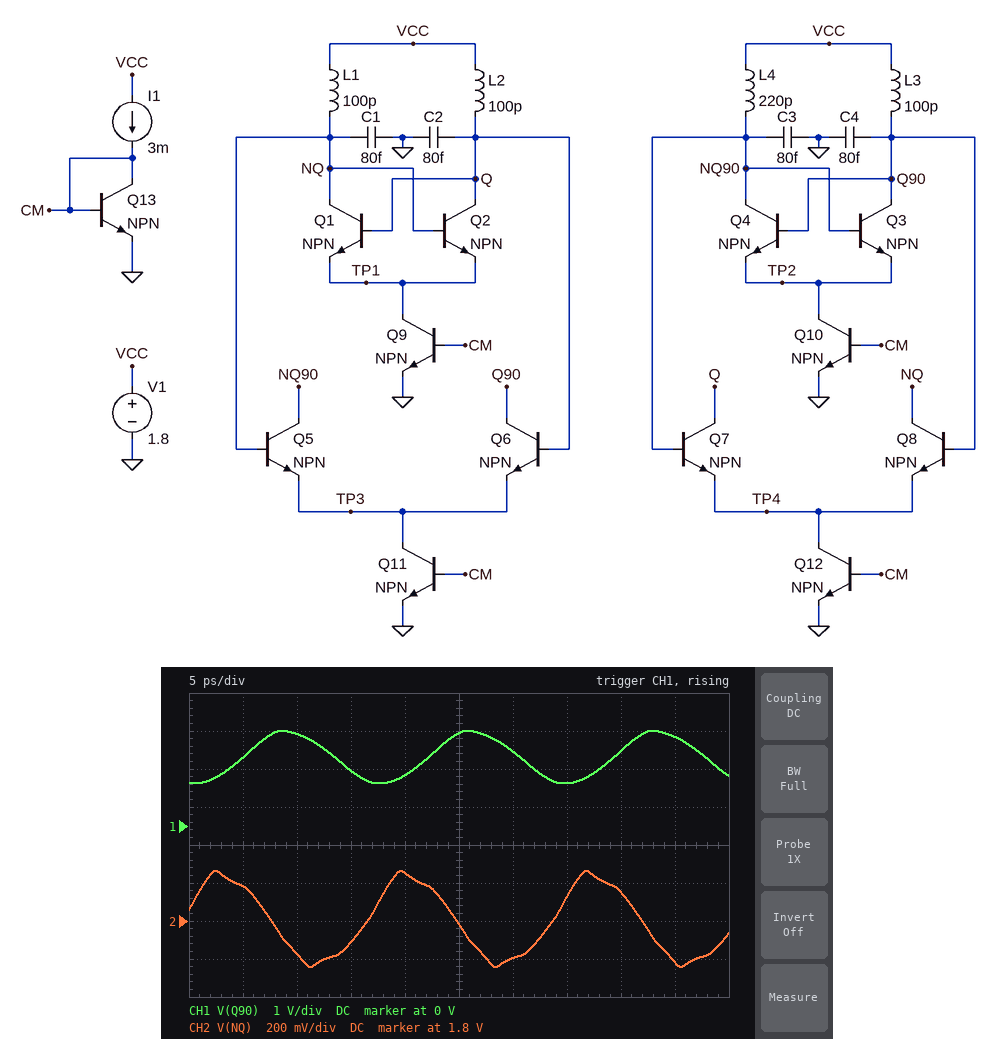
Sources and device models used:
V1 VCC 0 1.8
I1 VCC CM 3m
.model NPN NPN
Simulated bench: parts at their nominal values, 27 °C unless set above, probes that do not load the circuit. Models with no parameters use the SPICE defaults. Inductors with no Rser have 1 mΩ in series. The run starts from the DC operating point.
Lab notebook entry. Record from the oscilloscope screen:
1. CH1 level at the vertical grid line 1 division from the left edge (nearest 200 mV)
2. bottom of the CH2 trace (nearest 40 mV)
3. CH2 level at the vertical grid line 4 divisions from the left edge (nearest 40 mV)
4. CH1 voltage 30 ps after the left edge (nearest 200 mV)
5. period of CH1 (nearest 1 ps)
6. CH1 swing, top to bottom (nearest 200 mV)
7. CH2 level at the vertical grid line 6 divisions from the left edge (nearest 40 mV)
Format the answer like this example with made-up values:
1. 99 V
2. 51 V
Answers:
1. 1.8 V
2. 1.56 V
3. 2.04 V
4. 2.0 V
5. 17 ps
6. 1.4 V
7. 1.60 V
